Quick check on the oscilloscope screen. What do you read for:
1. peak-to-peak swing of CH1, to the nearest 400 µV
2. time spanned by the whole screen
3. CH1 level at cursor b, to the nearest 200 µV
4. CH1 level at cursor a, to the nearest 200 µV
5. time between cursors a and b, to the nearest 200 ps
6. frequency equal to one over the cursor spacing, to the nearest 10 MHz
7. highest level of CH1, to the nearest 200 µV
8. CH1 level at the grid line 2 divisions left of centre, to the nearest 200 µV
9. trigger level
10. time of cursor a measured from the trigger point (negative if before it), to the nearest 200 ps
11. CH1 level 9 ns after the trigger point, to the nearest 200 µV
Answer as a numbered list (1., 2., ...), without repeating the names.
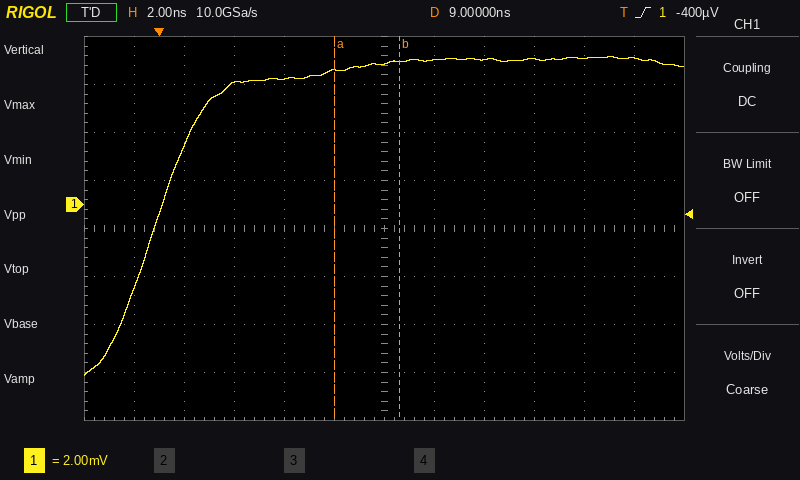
1. 13.2 mV
2. 24 ns
3. 6.0 mV
4. 5.6 mV
5. 2.6 ns
6. 380 MHz
7. 6.2 mV
8. 5.2 mV
9. -400 µV
10. +7.0 ns
11. 5.8 mV
